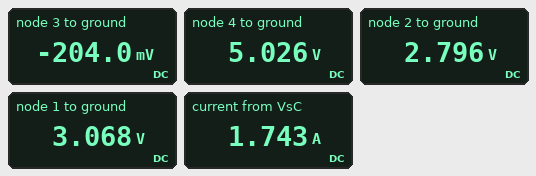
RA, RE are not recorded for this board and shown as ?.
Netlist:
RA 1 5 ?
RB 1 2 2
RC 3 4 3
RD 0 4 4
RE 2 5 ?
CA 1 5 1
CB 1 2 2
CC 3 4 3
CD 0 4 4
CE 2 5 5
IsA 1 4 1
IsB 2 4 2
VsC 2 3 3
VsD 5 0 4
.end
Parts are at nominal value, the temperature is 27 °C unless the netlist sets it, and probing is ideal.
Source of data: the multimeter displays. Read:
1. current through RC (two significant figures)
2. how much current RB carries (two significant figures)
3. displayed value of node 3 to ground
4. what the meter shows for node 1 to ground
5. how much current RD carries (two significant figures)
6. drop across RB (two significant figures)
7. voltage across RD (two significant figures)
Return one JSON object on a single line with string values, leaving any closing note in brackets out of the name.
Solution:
{"current through RC": "1.7 A", "how much current RB carries": "140 mA", "displayed value of node 3 to ground": "-204.0 mV", "what the meter shows for node 1 to ground": "3.068 V", "how much current RD carries": "1.3 A", "drop across RB": "270 mV", "voltage across RD": "5.0 V"}
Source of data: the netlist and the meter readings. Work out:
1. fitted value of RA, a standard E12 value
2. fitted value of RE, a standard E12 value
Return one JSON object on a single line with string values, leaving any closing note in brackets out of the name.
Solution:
{"fitted value of RA, a standard E12 value": "0.82 Ω", "fitted value of RE, a standard E12 value": "10 Ω"}
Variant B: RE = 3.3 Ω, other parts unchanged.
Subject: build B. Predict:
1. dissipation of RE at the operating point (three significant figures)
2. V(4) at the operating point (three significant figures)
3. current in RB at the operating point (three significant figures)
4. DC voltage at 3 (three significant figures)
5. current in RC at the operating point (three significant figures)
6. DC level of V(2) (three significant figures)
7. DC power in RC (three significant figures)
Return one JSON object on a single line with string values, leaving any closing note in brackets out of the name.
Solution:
{"dissipation of RE at the operating point": "245 mW", "V(4) at the operating point": "5.20 V", "current in RB at the operating point": "27.9 mA", "DC voltage at 3": "101 mV", "current in RC at the operating point": "1.70 A", "DC level of V(2)": "3.10 V", "DC power in RC": "8.67 W"}
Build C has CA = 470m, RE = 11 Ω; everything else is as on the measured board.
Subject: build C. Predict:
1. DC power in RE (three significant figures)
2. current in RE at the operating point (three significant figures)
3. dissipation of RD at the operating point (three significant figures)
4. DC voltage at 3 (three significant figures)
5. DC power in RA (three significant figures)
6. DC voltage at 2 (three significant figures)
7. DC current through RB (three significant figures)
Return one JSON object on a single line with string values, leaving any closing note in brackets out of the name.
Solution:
{"DC power in RE": "136 mW", "current in RE at the operating point": "111 mA", "dissipation of RD at the operating point": "6.29 W", "DC voltage at 3": "-223 mV", "DC power in RA": "1.07 W", "DC voltage at 2": "2.78 V", "DC current through RB": "143 mA"}
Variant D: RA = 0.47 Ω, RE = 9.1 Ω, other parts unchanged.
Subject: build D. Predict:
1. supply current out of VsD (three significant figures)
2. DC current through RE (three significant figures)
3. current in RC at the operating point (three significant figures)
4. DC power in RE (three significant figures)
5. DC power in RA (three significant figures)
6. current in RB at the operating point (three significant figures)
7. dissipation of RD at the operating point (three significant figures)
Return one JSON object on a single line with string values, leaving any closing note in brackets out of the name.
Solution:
{"supply current out of VsD": "1.29 A", "DC current through RE": "103 mA", "current in RC at the operating point": "1.71 A", "DC power in RE": "97.3 mW", "DC power in RA": "666 mW", "current in RB at the operating point": "191 mA", "dissipation of RD at the operating point": "6.70 W"}
